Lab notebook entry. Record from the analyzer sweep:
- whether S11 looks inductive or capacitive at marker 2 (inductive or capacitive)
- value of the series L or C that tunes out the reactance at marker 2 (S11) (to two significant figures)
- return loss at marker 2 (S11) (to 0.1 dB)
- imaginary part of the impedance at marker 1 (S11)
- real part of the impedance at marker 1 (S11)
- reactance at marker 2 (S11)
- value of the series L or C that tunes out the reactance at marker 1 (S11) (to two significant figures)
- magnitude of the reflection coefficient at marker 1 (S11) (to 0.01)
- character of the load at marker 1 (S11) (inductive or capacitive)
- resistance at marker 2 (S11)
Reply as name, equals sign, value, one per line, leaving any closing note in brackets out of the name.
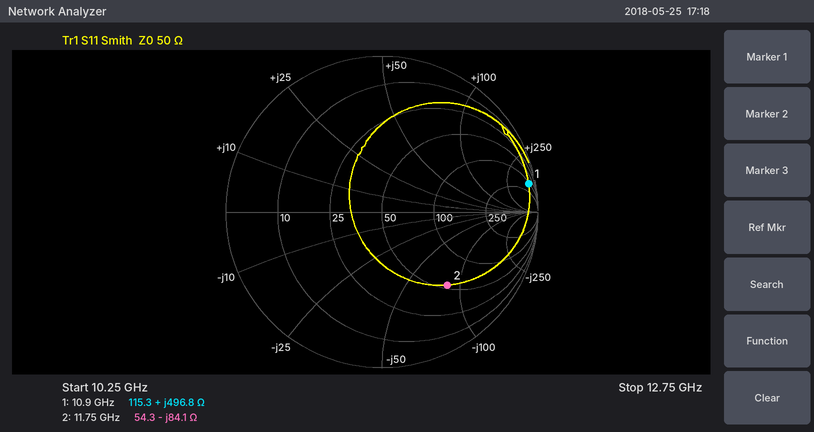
whether S11 looks inductive or capacitive at marker 2 = capacitive
value of the series L or C that tunes out the reactance at marker 2 (S11) = 1.1 nH
return loss at marker 2 (S11) = 4.0 dB
imaginary part of the impedance at marker 1 = +496.8 Ω
real part of the impedance at marker 1 = 115.3 Ω
reactance at marker 2 = -84.1 Ω
value of the series L or C that tunes out the reactance at marker 1 (S11) = 29 fF
magnitude of the reflection coefficient at marker 1 (S11) = 0.96
character of the load at marker 1 (S11) = inductive
resistance at marker 2 = 54.3 Ω
